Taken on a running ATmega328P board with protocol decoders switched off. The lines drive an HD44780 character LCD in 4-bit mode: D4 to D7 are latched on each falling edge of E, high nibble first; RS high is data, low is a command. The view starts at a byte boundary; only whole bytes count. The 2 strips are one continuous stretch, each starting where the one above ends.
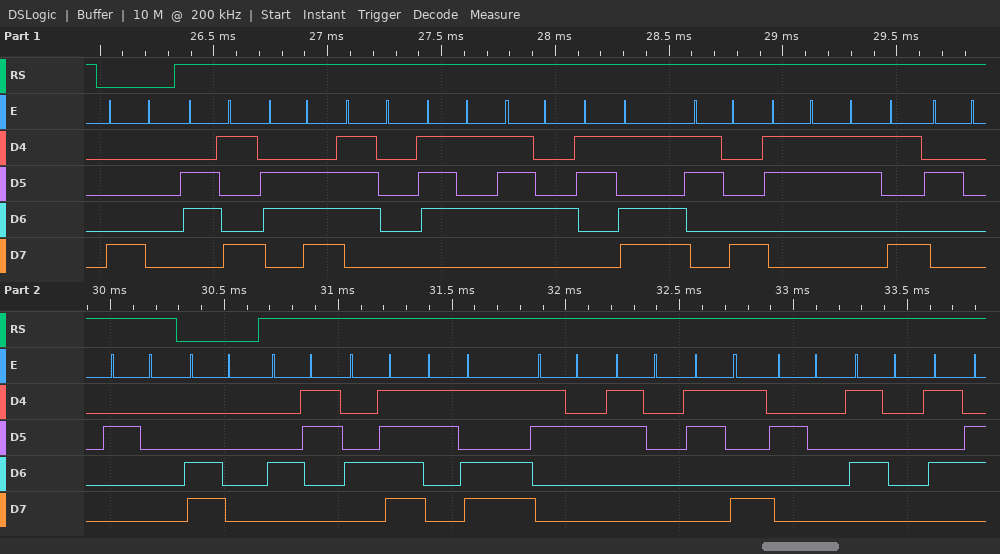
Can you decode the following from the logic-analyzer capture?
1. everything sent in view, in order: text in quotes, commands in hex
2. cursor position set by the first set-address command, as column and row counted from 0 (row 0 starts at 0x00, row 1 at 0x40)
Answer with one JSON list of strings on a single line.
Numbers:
["0x80 \"input=839  \" 0xC0 \"CO=209 PV\"", "column 0, row 0"]
